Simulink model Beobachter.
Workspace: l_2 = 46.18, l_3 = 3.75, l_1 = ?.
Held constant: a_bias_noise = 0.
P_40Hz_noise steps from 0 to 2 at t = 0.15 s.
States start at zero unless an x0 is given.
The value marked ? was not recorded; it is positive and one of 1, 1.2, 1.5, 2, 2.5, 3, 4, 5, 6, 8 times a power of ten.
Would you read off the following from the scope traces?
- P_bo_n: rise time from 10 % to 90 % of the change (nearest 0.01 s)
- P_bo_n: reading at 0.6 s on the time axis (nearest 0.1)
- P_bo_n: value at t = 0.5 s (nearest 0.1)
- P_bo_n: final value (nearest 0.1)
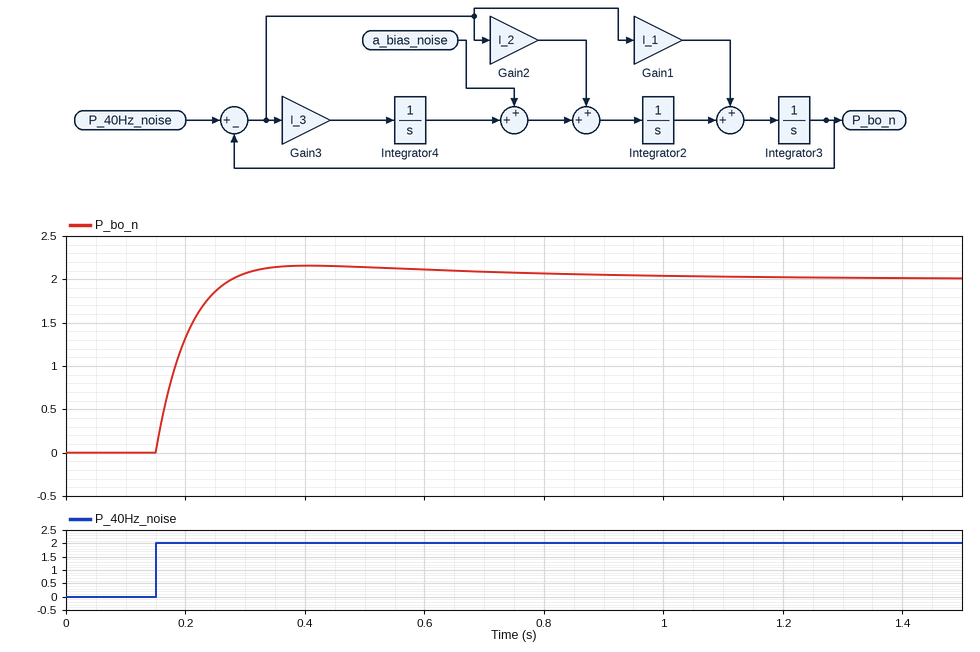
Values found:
0.09 s
2.1
2.1
2.0
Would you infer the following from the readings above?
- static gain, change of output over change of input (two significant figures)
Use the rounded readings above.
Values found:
1.0
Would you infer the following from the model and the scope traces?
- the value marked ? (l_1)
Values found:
20
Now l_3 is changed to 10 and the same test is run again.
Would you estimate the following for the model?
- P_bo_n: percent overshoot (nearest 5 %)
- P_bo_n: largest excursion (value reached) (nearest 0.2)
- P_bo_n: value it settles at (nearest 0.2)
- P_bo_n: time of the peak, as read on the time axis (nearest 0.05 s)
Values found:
10 %
2.2
2.0
0.40 s
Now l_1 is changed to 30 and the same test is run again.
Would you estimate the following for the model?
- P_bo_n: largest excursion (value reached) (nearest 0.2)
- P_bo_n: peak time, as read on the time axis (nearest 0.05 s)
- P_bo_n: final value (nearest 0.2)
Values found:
2.0
0.35 s
2.0
